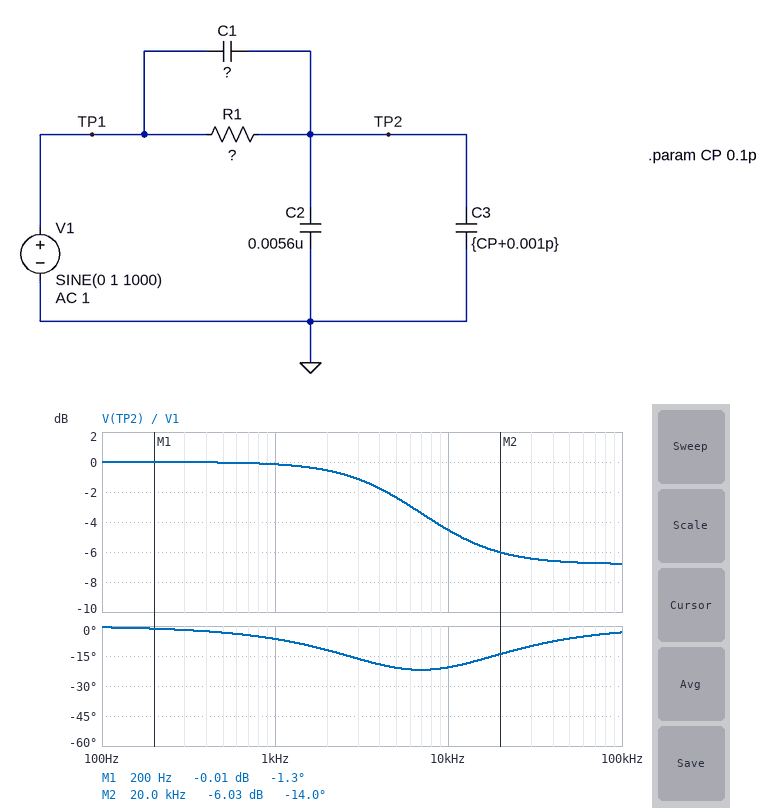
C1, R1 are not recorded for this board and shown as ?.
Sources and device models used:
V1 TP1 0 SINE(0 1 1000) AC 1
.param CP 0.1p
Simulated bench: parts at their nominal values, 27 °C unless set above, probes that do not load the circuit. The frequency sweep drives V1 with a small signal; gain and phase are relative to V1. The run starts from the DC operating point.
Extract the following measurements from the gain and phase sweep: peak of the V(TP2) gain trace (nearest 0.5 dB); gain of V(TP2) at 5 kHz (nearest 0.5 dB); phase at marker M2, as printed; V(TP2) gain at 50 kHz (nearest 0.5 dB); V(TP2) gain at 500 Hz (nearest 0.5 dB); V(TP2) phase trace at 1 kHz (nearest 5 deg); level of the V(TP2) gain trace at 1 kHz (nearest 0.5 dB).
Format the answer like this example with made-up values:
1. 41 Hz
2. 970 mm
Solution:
1. 0 dB
2. -2.5 dB
3. -14.0 deg
4. -6.5 dB
5. 0 dB
6. -5 deg
7. 0 dB
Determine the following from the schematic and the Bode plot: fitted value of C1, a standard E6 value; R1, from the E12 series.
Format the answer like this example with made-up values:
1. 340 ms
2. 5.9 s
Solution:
1. 4.7 nF
2. 3.3 kΩ
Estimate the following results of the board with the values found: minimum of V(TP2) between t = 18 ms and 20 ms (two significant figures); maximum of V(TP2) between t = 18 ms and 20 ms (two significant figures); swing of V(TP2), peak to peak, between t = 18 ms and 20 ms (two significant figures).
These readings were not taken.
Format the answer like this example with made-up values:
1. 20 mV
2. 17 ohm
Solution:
1. -980 mV
2. 980 mV
3. 2.0 V
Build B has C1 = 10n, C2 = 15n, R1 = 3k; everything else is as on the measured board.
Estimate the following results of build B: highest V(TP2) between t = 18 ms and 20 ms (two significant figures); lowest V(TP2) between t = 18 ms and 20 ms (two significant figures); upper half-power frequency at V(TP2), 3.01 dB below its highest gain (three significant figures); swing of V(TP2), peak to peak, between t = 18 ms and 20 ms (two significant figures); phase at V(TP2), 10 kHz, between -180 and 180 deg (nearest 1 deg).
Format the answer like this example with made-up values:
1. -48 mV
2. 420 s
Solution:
1. 920 mV
2. -920 mV
3. 2.57 kHz
4. 1.8 V
5. -16 deg
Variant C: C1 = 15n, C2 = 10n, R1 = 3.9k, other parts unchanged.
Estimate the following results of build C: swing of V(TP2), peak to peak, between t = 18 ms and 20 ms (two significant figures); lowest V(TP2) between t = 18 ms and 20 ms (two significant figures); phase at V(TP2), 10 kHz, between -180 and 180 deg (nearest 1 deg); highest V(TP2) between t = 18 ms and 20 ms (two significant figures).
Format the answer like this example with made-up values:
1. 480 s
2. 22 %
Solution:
1. 1.8 V
2. -910 mV
3. -6 deg
4. 910 mV
